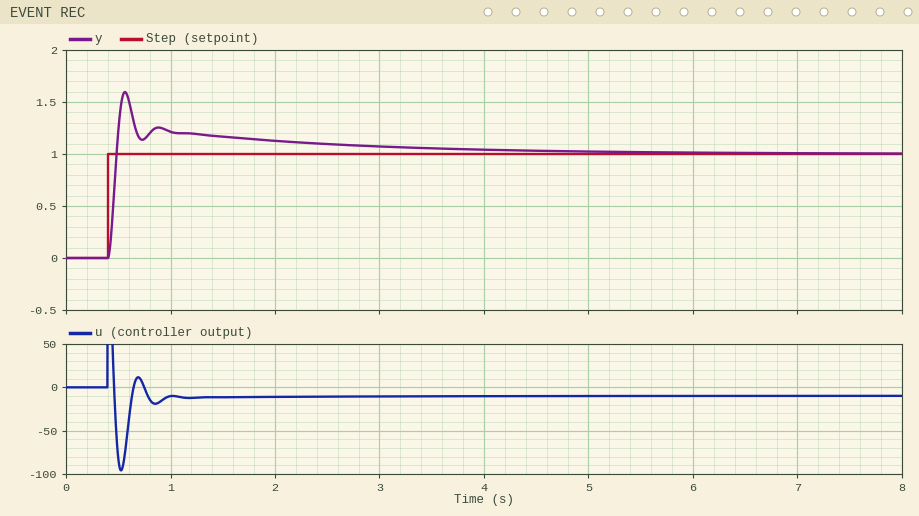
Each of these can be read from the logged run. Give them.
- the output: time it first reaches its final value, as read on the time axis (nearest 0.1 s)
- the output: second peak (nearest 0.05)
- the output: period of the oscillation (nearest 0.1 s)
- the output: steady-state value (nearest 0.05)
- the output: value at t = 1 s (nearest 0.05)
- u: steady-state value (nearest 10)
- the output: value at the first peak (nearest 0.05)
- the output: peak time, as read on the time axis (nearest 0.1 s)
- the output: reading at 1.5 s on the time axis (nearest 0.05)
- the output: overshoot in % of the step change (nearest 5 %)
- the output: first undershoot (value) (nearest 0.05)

0.5 s
1.25
0.3 s
1.00
1.20
-10
1.60
0.6 s
1.15
60 %
1.15
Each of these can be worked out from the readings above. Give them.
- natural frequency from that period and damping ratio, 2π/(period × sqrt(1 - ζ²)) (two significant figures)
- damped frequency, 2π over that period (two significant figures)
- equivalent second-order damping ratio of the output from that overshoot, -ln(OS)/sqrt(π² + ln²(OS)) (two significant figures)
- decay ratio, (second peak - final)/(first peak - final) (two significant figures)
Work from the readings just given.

21 rad/s
21 rad/s
0.16
0.42
